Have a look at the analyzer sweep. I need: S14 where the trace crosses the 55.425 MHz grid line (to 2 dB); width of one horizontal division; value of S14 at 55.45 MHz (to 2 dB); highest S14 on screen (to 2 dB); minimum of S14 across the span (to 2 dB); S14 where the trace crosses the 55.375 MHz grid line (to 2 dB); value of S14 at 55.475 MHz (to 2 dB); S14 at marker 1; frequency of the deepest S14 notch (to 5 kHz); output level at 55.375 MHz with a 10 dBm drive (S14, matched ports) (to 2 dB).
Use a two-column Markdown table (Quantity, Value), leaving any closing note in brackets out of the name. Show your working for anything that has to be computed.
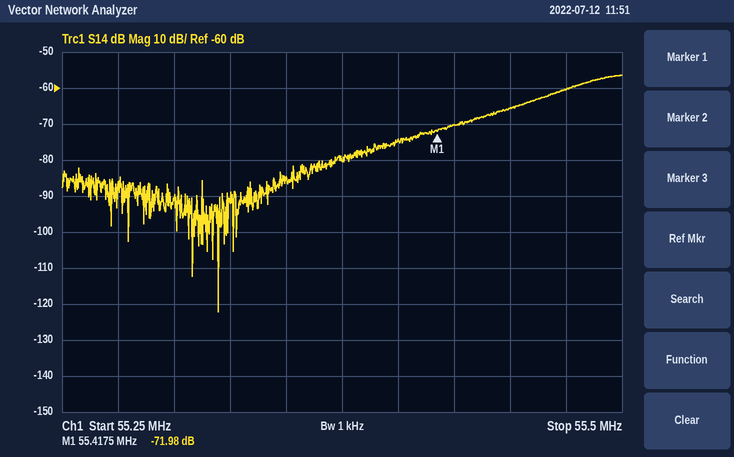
| Quantity | Value |
|---|---|
| S14 where the trace crosses the 55.425 MHz grid line | -70 dB |
| width of one horizontal division | 25 kHz |
| value of S14 at 55.45 MHz | -66 dB |
| highest S14 on screen | -56 dB |
| minimum of S14 across the span | -122 dB |
| S14 where the trace crosses the 55.375 MHz grid line | -80 dB |
| value of S14 at 55.475 MHz | -60 dB |
| S14 at marker 1 | -71.98 dB |
| frequency of the deepest S14 notch | 55.320 MHz |
| output level at 55.375 MHz with a 10 dBm drive (S14, matched ports) | 10 dBm + (-80 dB) = -70 dBm |
